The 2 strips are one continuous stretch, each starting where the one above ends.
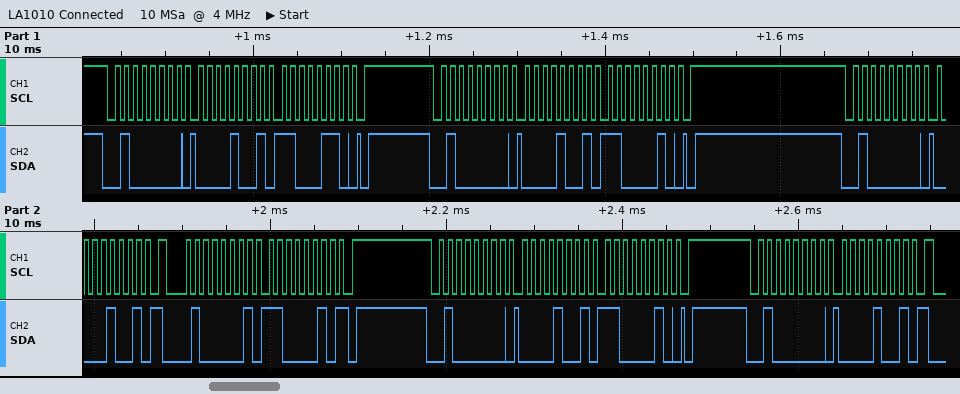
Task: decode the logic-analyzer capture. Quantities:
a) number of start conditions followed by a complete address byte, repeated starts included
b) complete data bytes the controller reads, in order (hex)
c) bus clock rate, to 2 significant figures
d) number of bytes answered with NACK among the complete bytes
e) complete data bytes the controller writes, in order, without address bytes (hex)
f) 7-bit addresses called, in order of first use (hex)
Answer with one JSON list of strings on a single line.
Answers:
["6", "C2", "100 kHz", "1", "09 C6 09 C2 09 09 C2 09", "0x20"]
